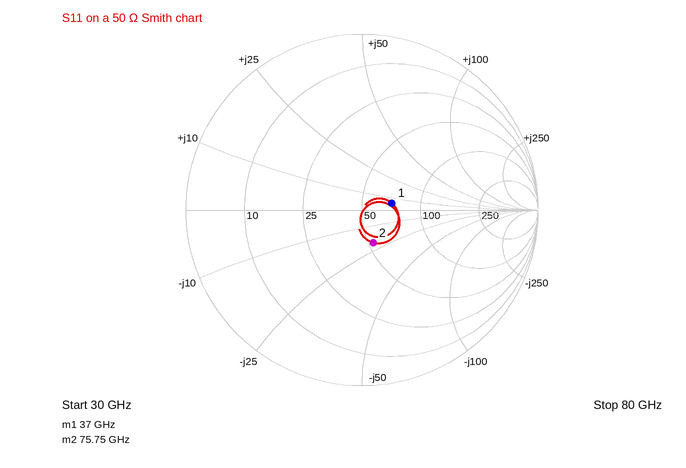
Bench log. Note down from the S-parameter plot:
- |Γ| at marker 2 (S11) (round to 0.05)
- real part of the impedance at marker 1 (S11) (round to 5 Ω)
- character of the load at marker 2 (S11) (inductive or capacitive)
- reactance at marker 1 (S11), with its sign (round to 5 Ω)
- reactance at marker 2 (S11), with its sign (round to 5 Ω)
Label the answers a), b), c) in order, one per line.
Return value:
a) 0.20
b) 70 Ω
c) capacitive
d) +5 Ω
e) -20 Ω
